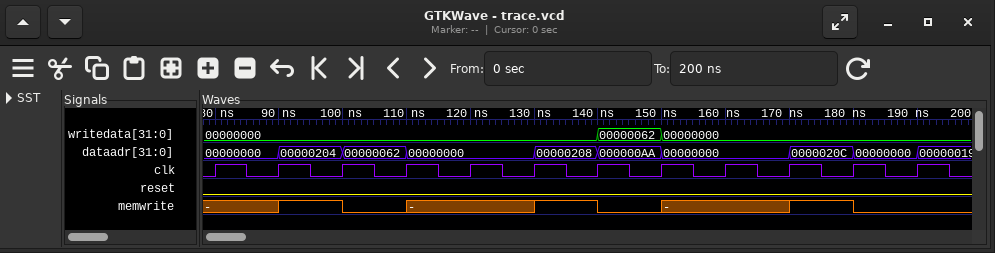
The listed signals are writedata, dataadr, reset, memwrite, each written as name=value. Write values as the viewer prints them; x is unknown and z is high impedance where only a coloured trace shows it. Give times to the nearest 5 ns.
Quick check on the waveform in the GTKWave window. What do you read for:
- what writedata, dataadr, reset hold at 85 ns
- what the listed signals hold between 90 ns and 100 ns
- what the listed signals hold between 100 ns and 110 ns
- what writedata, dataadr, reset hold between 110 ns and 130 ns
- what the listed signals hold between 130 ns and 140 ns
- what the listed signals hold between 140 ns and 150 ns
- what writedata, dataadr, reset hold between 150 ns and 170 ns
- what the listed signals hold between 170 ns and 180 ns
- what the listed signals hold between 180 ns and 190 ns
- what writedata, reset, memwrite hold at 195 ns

writedata=00000000, dataadr=00000000, reset=0
writedata=00000000, dataadr=00000204, reset=0, memwrite=1
writedata=00000000, dataadr=00000062, reset=0, memwrite=0
writedata=00000000, dataadr=00000000, reset=0
writedata=00000000, dataadr=00000208, reset=0, memwrite=1
writedata=00000062, dataadr=000000AA, reset=0, memwrite=0
writedata=00000000, dataadr=00000000, reset=0
writedata=00000000, dataadr=0000020C, reset=0, memwrite=1
writedata=00000000, dataadr=00000000, reset=0, memwrite=0
writedata=00000000, reset=0, memwrite=0
